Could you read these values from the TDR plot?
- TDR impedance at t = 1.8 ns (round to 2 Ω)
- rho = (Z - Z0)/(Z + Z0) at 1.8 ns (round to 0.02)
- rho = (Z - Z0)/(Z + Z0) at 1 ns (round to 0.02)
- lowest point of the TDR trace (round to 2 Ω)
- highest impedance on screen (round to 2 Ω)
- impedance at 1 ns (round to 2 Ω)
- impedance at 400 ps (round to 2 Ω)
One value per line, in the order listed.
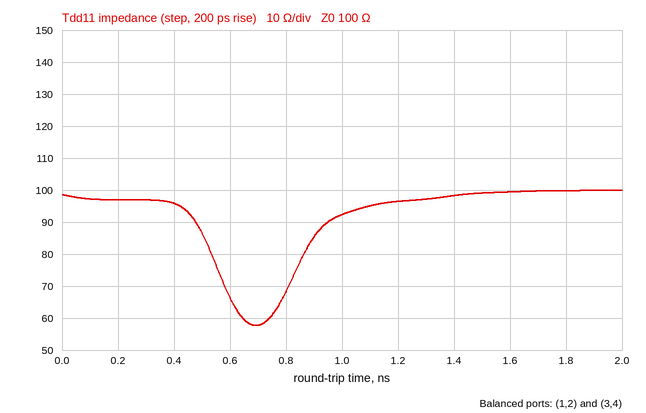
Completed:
100 Ω
0.00
-0.04
58 Ω
100 Ω
92 Ω
96 Ω
